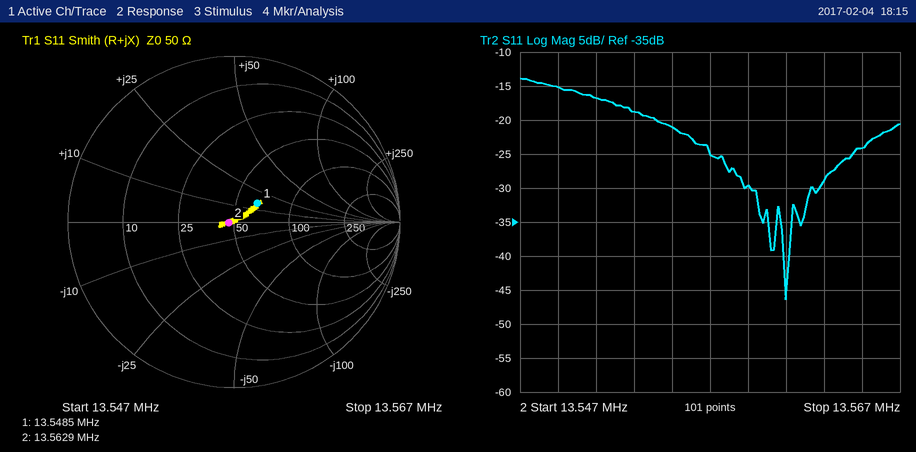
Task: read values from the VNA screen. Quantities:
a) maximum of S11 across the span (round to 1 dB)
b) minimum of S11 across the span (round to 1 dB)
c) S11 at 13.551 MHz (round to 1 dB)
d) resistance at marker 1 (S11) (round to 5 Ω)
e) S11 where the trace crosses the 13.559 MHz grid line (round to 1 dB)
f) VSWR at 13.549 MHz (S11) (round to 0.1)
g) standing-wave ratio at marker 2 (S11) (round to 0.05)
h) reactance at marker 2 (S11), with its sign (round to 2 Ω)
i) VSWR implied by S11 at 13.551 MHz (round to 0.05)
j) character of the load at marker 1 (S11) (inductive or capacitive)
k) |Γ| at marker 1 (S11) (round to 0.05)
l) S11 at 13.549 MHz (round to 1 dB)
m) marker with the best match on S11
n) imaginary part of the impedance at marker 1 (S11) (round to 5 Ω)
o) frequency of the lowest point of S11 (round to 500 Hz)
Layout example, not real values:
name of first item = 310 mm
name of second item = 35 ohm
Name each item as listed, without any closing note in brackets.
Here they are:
maximum of S11 across the span = -14 dB
minimum of S11 across the span = -46 dB
S11 at 13.551 MHz = -17 dB
resistance at marker 1 (S11) = 65 Ω
S11 where the trace crosses the 13.559 MHz grid line = -30 dB
VSWR at 13.549 MHz (S11) = 1.4
standing-wave ratio at marker 2 (S11) = 1.05
reactance at marker 2 (S11), with its sign = 0 Ω
VSWR implied by S11 at 13.551 MHz = 1.35
character of the load at marker 1 (S11) = inductive
|Γ| at marker 1 (S11) = 0.20
S11 at 13.549 MHz = -15 dB
marker with the best match on S11 = marker 2
imaginary part of the impedance at marker 1 (S11) = +15 Ω
frequency of the lowest point of S11 = 13.5610 MHz
